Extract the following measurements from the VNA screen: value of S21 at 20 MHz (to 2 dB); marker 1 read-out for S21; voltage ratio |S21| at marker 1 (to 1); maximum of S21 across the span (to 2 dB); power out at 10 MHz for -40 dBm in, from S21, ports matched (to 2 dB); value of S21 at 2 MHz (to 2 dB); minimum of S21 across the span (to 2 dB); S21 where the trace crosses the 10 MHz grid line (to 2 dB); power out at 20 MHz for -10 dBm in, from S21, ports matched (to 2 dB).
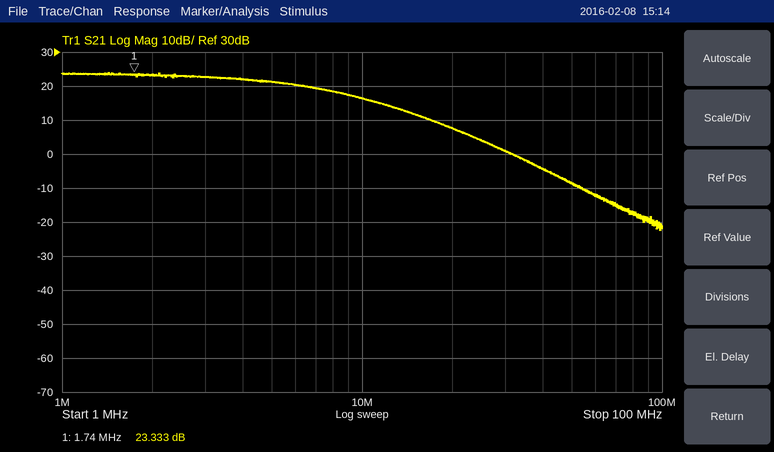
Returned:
8 dB
23.333 dB
15
24 dB
-24 dBm
24 dB
-22 dB
16 dB
-2 dBm
